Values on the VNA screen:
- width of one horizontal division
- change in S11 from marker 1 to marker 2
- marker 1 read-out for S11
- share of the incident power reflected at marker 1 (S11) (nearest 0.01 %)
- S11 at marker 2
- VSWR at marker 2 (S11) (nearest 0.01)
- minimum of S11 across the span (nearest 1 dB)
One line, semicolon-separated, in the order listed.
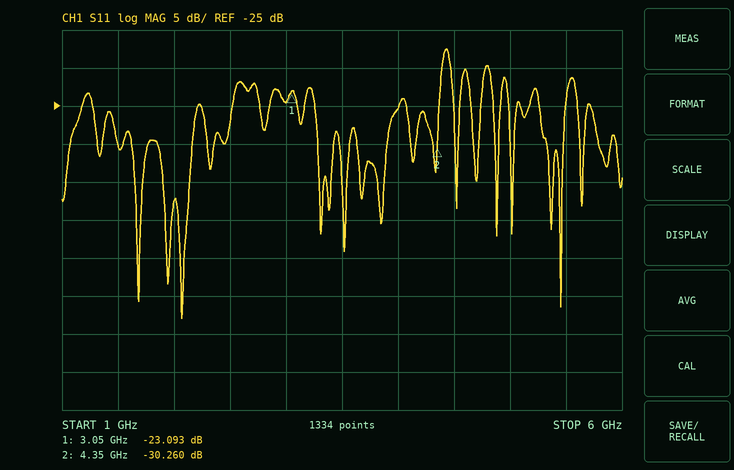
500 MHz; -7.167 dB; -23.093 dB; 0.49 %; -30.260 dB; 1.06; -53 dB
